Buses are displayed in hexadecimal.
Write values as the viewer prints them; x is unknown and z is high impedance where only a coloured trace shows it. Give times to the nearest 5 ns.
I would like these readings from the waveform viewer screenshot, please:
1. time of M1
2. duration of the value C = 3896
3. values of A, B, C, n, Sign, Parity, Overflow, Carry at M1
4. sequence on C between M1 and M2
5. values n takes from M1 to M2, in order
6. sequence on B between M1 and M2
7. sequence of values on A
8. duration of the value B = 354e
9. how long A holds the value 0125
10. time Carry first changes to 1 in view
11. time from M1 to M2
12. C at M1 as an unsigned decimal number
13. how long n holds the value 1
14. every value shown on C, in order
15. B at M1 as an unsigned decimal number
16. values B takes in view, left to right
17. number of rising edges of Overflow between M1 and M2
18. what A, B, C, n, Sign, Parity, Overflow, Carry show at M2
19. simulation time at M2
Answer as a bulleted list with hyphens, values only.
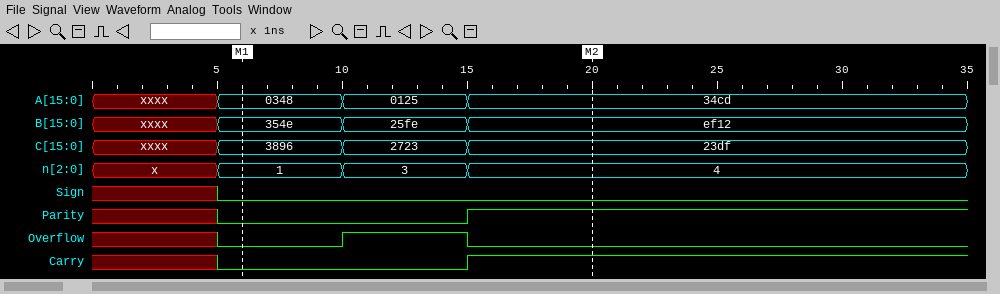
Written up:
- 5 ns
- 5 ns
- A=0348, B=354e, C=3896, n=1, Sign=0, Parity=0, Overflow=0, Carry=0
- 3896, 2723, 23df
- 1, 3, 4
- 354e, 25fe, ef12
- xxxx, 0348, 0125, 34cd
- 5 ns
- 5 ns
- 15 ns
- 15 ns
- 14486
- 5 ns
- xxxx, 3896, 2723, 23df
- 13646
- xxxx, 354e, 25fe, ef12
- 1
- A=34cd, B=ef12, C=23df, n=4, Sign=0, Parity=1, Overflow=0, Carry=1
- 20 ns
